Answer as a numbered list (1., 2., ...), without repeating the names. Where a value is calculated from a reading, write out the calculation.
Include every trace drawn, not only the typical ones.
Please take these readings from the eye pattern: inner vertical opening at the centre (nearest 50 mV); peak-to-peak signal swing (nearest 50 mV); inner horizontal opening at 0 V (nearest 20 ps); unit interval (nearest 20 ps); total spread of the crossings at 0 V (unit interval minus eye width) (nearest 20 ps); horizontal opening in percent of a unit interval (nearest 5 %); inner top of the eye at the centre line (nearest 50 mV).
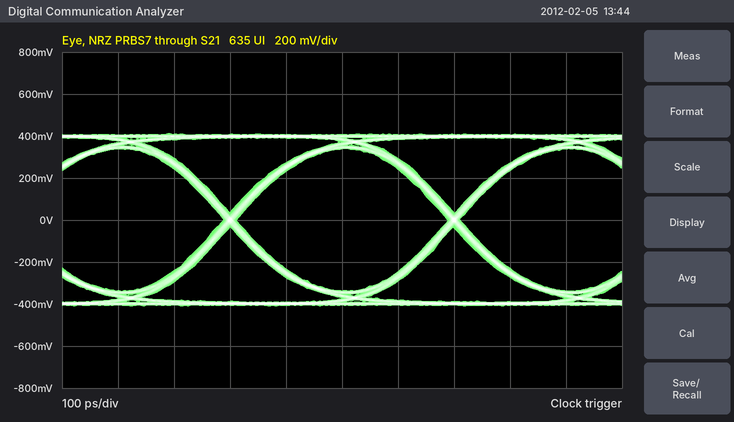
1. 700 mV
2. 800 mV
3. 380 ps
4. 400 ps
5. 20 ps
6. 380 ps / 400 ps ≈ 95 %
7. 350 mV
